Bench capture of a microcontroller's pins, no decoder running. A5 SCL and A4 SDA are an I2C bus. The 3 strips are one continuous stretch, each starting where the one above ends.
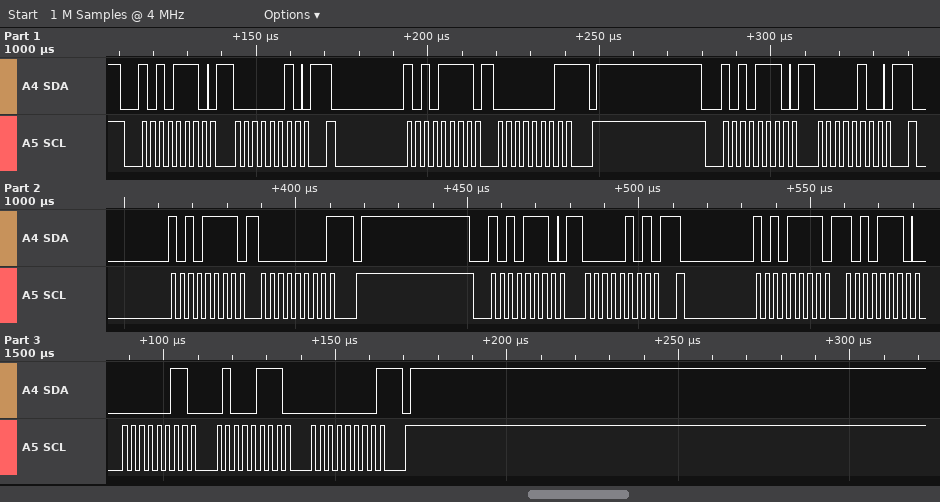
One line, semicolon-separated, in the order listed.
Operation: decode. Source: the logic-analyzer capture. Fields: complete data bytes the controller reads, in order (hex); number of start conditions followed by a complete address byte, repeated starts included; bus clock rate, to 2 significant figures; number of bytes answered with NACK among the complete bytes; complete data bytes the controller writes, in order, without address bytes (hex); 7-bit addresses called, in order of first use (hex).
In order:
01 00 AE 03 47 00; 6; 400 kHz; 3; 02 04 05; 0x57
